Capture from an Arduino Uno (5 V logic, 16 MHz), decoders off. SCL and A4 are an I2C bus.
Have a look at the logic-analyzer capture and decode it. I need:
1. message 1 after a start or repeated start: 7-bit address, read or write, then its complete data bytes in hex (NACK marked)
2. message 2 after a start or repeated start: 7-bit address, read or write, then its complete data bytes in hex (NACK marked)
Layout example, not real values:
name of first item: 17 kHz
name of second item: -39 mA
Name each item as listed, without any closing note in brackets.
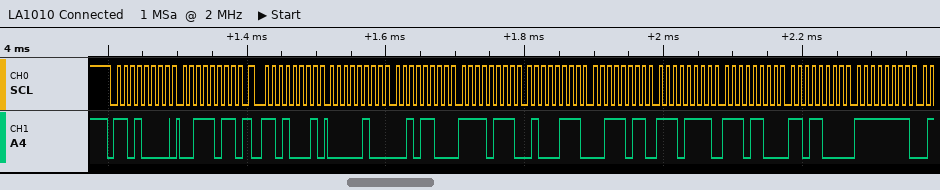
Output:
message 1 after a start or repeated start: 7-bit address, read or write, then its complete data bytes in hex: 0x68 write: 3B
message 2 after a start or repeated start: 7-bit address, read or write, then its complete data bytes in hex: 0x68 read: 04 2C F7 47 3B EF EC D8 FF
